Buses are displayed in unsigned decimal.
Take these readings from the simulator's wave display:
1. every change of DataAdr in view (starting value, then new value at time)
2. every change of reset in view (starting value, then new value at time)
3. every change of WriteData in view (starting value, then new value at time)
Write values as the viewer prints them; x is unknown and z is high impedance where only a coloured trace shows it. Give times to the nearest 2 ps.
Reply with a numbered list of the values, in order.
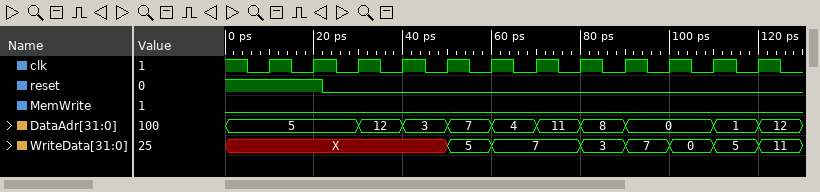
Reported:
1. 5, 12 at 30 ps, 3 at 40 ps, 7 at 50 ps, 4 at 60 ps, 11 at 70 ps, 8 at 80 ps, 0 at 90 ps, 1 at 110 ps, 12 at 120 ps
2. 1, 0 at 22 ps
3. X, 5 at 50 ps, 7 at 60 ps, 3 at 80 ps, 7 at 90 ps, 0 at 100 ps, 5 at 110 ps, 11 at 120 ps
